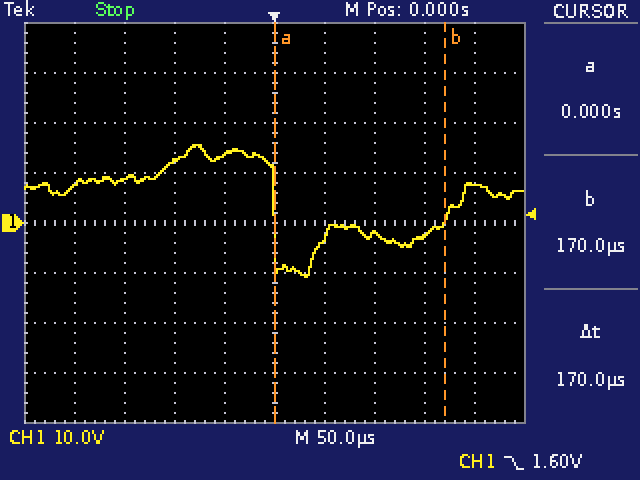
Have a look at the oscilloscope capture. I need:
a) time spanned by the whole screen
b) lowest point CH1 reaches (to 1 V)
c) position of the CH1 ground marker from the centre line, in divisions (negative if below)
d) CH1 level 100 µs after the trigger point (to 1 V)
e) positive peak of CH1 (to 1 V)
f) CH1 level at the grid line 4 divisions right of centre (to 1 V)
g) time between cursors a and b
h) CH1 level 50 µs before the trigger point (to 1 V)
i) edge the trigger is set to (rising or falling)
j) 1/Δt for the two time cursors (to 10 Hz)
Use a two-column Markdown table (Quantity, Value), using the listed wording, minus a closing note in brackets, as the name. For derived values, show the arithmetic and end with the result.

| Quantity | Value |
|---|---|
| time spanned by the whole screen | 500 µs |
| lowest point CH1 reaches | -11 V |
| position of the CH1 ground marker from the centre line, in divisions | 0.0 div |
| CH1 level 100 µs after the trigger point | -2 V |
| positive peak of CH1 | 16 V |
| CH1 level at the grid line 4 divisions right of centre | 8 V |
| time between cursors a and b | 170 µs |
| CH1 level 50 µs before the trigger point | 14 V |
| edge the trigger is set to | falling |
| 1/Δt for the two time cursors | 1 / 170 µs ≈ 5.88 kHz |
